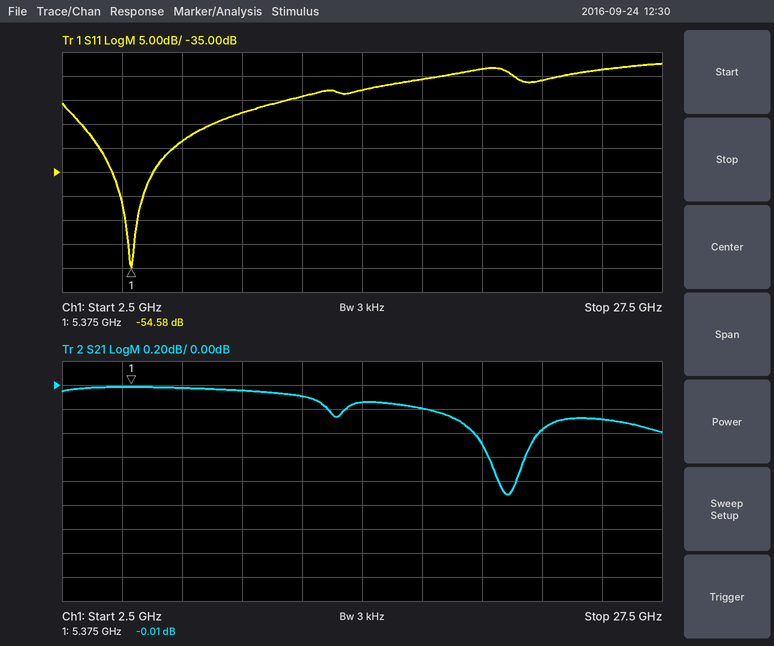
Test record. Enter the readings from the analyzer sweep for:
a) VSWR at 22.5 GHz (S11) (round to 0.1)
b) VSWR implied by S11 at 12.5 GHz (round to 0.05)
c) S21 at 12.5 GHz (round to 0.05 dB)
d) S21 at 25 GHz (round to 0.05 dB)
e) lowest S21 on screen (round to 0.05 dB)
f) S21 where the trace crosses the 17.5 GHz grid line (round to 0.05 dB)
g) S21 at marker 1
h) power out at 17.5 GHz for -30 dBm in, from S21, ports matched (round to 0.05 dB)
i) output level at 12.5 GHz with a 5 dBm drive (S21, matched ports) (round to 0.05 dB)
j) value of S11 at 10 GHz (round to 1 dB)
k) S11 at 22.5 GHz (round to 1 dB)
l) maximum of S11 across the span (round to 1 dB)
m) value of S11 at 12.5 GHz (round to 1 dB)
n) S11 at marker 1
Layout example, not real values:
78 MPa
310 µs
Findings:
1.4
1.25
-0.10 dB
-0.30 dB
-0.90 dB
-0.20 dB
-0.01 dB
-30.20 dBm
4.90 dBm
-23 dB
-16 dB
-12 dB
-19 dB
-54.58 dB
